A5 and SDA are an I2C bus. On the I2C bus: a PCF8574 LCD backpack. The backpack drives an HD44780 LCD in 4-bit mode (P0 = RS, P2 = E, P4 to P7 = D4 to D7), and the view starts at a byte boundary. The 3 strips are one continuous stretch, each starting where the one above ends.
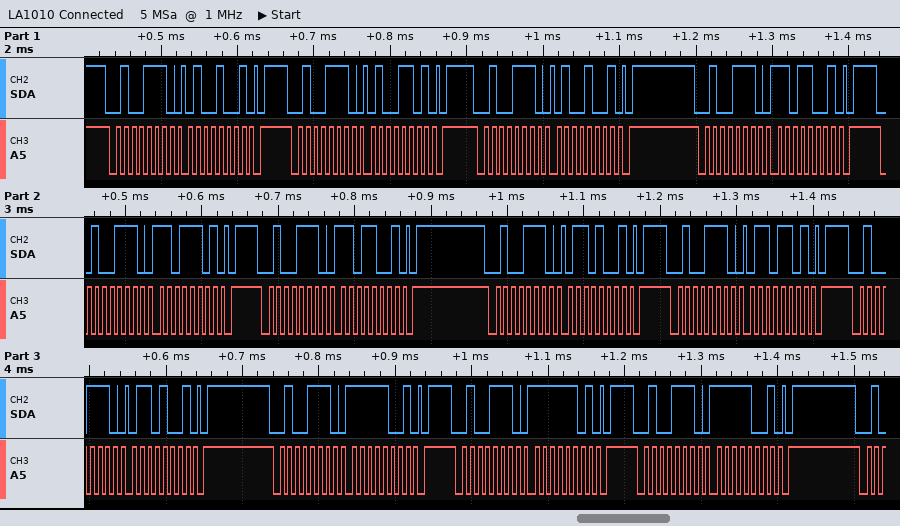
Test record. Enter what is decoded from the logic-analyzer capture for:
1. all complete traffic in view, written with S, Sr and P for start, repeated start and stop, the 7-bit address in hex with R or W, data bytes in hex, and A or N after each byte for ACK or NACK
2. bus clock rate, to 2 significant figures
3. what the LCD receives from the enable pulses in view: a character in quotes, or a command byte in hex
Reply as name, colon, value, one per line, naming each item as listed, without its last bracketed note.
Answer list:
all complete traffic in view, written with S, Sr and P for start, repeated start and stop, the 7-bit address in hex with R or W, data bytes in hex, and A or N after each byte for ACK or NACK: S 27W A 49 A P S 27W A 4D A P S 27W A 49 A P S 27W A D9 A P S 27W A DD A P S 27W A D9 A P S 27W A 69 A P S 27W A 6D A P S 27W A 69 A P S 27W A F9 A P S 27W A FD A P S 27W A F9 A P
bus clock rate, to 2 significant figures: 100 kHz
what the LCD receives from the enable pulses in view: a character in quotes, or a command byte in hex: 'M' 'o'
